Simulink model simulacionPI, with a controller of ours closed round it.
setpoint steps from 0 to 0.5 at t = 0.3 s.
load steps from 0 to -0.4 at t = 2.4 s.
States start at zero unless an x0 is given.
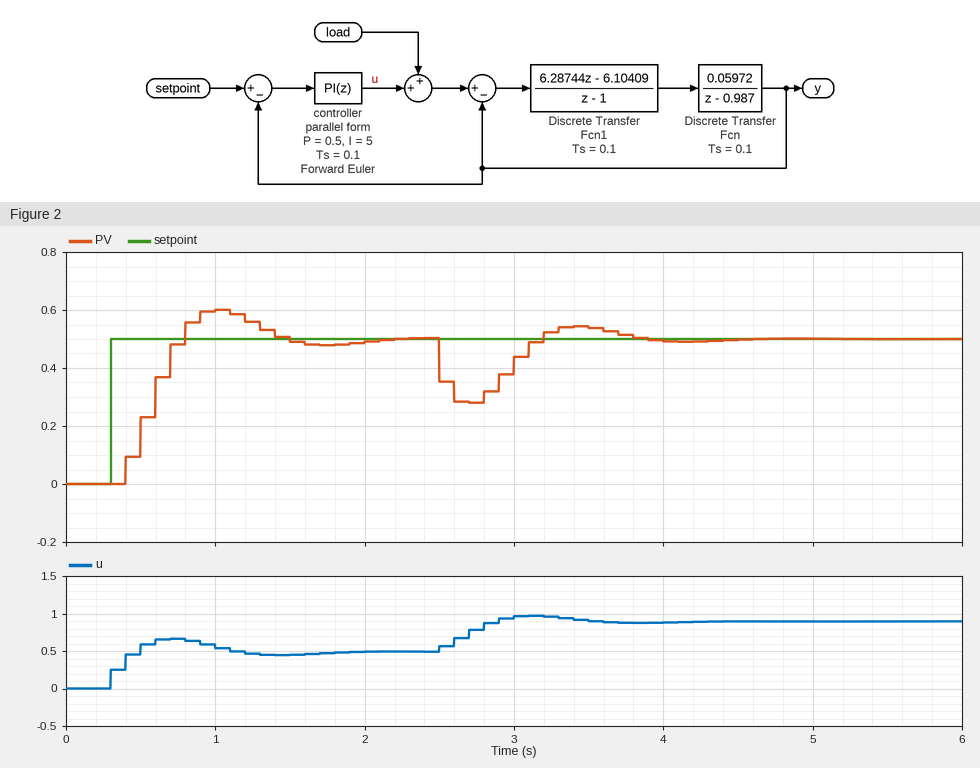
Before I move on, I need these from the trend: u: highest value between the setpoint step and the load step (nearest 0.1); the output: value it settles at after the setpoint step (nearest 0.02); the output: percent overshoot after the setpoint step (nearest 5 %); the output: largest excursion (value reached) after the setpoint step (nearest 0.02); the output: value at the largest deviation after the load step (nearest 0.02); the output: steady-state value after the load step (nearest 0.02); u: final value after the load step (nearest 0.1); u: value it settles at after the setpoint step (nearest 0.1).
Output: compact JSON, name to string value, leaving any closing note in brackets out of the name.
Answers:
{"u: highest value between the setpoint step and the load step": "0.7", "the output: value it settles at after the setpoint step": "0.50", "the output: percent overshoot after the setpoint step": "20 %", "the output: largest excursion (value reached) after the setpoint step": "0.60", "the output: value at the largest deviation after the load step": "0.28", "the output: steady-state value after the load step": "0.50", "u: final value after the load step": "0.9", "u: value it settles at after the setpoint step": "0.5"}
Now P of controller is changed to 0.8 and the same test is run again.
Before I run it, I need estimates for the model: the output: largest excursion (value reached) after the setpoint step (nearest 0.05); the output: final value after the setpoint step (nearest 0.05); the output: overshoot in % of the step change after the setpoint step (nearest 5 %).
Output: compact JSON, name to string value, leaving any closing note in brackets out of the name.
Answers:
{"the output: largest excursion (value reached) after the setpoint step": "0.55", "the output: final value after the setpoint step": "0.50", "the output: overshoot in % of the step change after the setpoint step": "10 %"}
